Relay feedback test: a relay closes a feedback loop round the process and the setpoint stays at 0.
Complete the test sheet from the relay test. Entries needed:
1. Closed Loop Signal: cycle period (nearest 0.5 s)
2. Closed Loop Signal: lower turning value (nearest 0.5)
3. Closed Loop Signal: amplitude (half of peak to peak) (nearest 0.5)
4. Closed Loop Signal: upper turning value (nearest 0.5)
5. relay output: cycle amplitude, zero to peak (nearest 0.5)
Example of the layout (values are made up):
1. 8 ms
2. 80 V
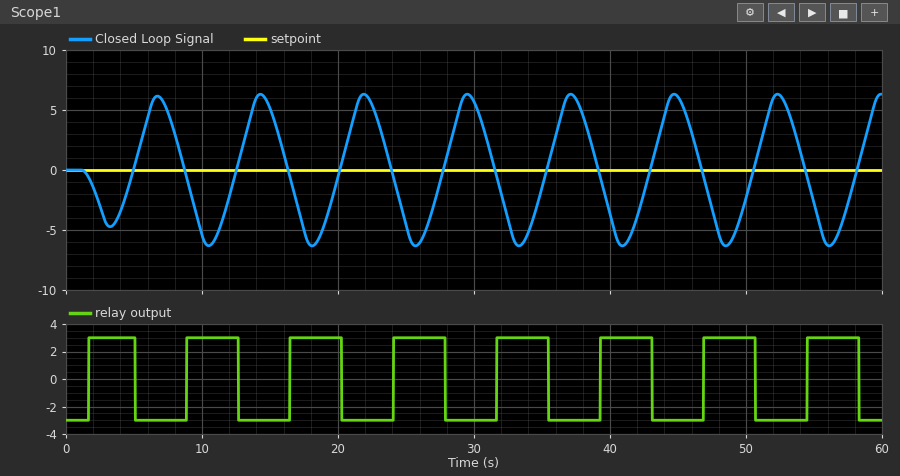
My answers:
1. 7.5 s
2. -6.5
3. 6.5
4. 6.5
5. 3.0
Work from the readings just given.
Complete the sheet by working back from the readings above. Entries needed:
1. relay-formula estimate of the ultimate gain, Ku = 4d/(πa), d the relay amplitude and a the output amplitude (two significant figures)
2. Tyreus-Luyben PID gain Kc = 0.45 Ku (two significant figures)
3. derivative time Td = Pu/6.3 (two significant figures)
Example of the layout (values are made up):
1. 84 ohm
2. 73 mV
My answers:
1. 0.59
2. 0.27
3. 1.2 s
